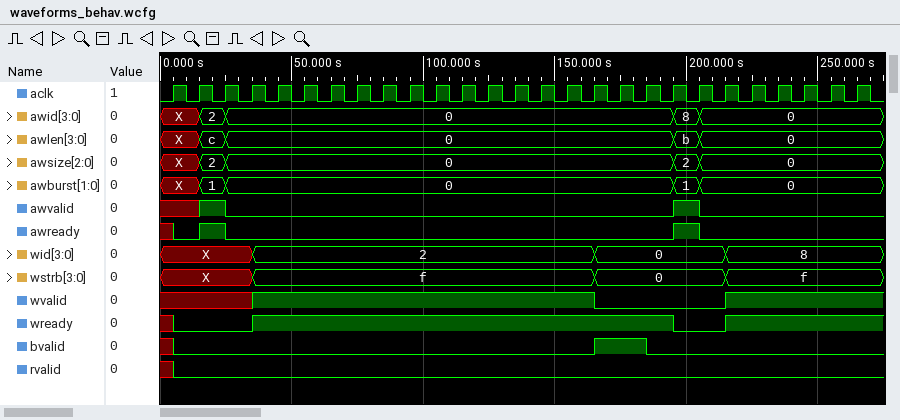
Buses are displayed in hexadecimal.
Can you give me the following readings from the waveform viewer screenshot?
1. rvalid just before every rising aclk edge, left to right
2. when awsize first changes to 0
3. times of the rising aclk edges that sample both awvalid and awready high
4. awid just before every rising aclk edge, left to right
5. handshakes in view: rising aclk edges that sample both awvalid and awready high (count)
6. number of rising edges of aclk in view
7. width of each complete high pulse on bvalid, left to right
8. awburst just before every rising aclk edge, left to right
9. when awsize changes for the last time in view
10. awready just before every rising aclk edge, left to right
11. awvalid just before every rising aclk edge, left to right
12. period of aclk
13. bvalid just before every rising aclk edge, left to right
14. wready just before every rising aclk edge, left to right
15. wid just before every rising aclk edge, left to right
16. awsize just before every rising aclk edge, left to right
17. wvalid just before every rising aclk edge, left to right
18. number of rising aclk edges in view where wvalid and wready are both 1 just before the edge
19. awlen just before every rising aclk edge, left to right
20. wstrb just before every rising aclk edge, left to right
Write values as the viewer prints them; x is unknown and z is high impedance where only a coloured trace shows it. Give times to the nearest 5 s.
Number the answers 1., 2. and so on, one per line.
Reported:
1. x 0 0 0 0 0 0 0 0 0 0 0 0 0 0 0 0 0 0 0 0 0 0 0 0 0 0
2. 25 s
3. 25 s, 205 s
4. X, X, 2, 0, 0, 0, 0, 0, 0, 0, 0, 0, 0, 0, 0, 0, 0, 0, 0, 0, 8, 0, 0, 0, 0, 0, 0
5. 2
6. 27
7. 20 s
8. X, X, 1, 0, 0, 0, 0, 0, 0, 0, 0, 0, 0, 0, 0, 0, 0, 0, 0, 0, 1, 0, 0, 0, 0, 0, 0
9. 205 s
10. x 0 1 0 0 0 0 0 0 0 0 0 0 0 0 0 0 0 0 0 1 0 0 0 0 0 0
11. x x 1 0 0 0 0 0 0 0 0 0 0 0 0 0 0 0 0 0 1 0 0 0 0 0 0
12. 10 s
13. x 0 0 0 0 0 0 0 0 0 0 0 0 0 0 0 0 1 1 0 0 0 0 0 0 0 0
14. x 0 0 0 1 1 1 1 1 1 1 1 1 1 1 1 1 1 1 1 0 0 1 1 1 1 1
15. X, X, X, X, 2, 2, 2, 2, 2, 2, 2, 2, 2, 2, 2, 2, 2, 0, 0, 0, 0, 0, 8, 8, 8, 8, 8
16. X, X, 2, 0, 0, 0, 0, 0, 0, 0, 0, 0, 0, 0, 0, 0, 0, 0, 0, 0, 2, 0, 0, 0, 0, 0, 0
17. x x x x 1 1 1 1 1 1 1 1 1 1 1 1 1 0 0 0 0 0 1 1 1 1 1
18. 18
19. X, X, c, 0, 0, 0, 0, 0, 0, 0, 0, 0, 0, 0, 0, 0, 0, 0, 0, 0, b, 0, 0, 0, 0, 0, 0
20. X, X, X, X, f, f, f, f, f, f, f, f, f, f, f, f, f, 0, 0, 0, 0, 0, f, f, f, f, f
